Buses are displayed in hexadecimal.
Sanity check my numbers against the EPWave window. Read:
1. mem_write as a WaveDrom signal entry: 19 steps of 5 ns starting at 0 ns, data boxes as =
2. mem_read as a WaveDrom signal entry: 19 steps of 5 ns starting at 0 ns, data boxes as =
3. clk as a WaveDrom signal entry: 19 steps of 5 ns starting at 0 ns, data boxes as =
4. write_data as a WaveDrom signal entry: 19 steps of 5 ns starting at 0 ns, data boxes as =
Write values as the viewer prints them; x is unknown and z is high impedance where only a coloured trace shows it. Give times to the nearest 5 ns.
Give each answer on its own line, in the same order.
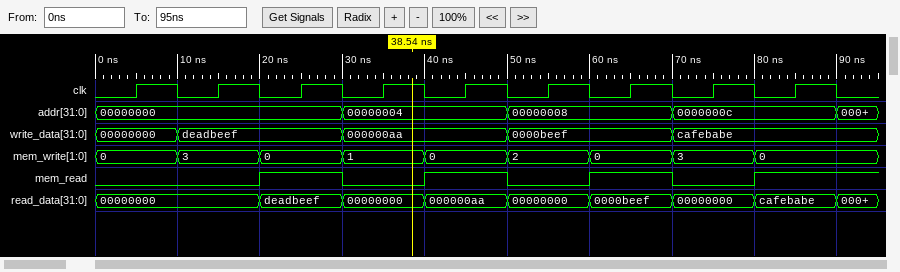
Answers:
{name: 'mem_write', wave: '=.=.=.=.=.=.=.=.=..', data: '0 3 0 1 0 2 0 3 0'}
{name: 'mem_read', wave: '0...1.0.1.0.1.0.1..'}
{name: 'clk', wave: '0101010101010101010'}
{name: 'write_data', wave: '=.=...=...=...=....', data: '00000000 deadbeef 000000aa 0000beef cafebabe'}
